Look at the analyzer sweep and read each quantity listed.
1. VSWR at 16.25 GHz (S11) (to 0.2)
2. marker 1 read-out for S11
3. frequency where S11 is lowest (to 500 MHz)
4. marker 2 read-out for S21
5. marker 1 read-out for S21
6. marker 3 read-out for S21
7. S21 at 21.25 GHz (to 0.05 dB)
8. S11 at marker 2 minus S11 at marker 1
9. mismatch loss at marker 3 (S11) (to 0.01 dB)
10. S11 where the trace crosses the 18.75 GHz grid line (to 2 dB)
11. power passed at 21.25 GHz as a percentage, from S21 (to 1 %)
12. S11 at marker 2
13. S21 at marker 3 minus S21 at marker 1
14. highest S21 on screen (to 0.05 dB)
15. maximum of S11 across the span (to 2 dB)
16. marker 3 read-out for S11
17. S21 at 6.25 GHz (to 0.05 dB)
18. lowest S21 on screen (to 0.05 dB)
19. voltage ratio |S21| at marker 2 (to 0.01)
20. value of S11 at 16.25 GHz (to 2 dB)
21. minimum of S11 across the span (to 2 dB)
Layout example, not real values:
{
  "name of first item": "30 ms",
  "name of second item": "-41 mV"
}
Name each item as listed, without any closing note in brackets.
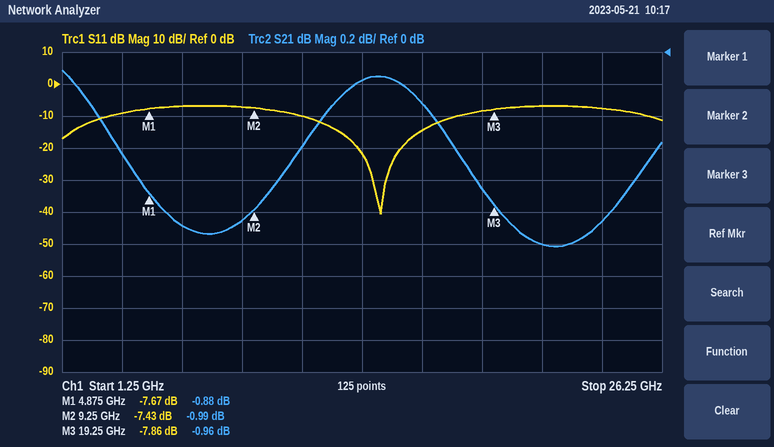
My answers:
{
  "VSWR at 16.25 GHz (S11)": "1.4",
  "marker 1 read-out for S11": "-7.67 dB",
  "frequency where S11 is lowest": "14.5 GHz",
  "marker 2 read-out for S21": "-0.99 dB",
  "marker 1 read-out for S21": "-0.88 dB",
  "marker 3 read-out for S21": "-0.96 dB",
  "S21 at 21.25 GHz": "-1.20 dB",
  "S11 at marker 2 minus S11 at marker 1": "0.24 dB",
  "mismatch loss at marker 3 (S11)": "0.78 dB",
  "S11 where the trace crosses the 18.75 GHz grid line": "-8 dB",
  "power passed at 21.25 GHz as a percentage, from S21": "76 %",
  "S11 at marker 2": "-7.43 dB",
  "S21 at marker 3 minus S21 at marker 1": "-0.08 dB",
  "highest S21 on screen": "-0.10 dB",
  "maximum of S11 across the span": "-6 dB",
  "marker 3 read-out for S11": "-7.86 dB",
  "S21 at 6.25 GHz": "-1.10 dB",
  "lowest S21 on screen": "-1.20 dB",
  "voltage ratio |S21| at marker 2": "0.89",
  "value of S11 at 16.25 GHz": "-14 dB",
  "minimum of S11 across the span": "-40 dB"
}
